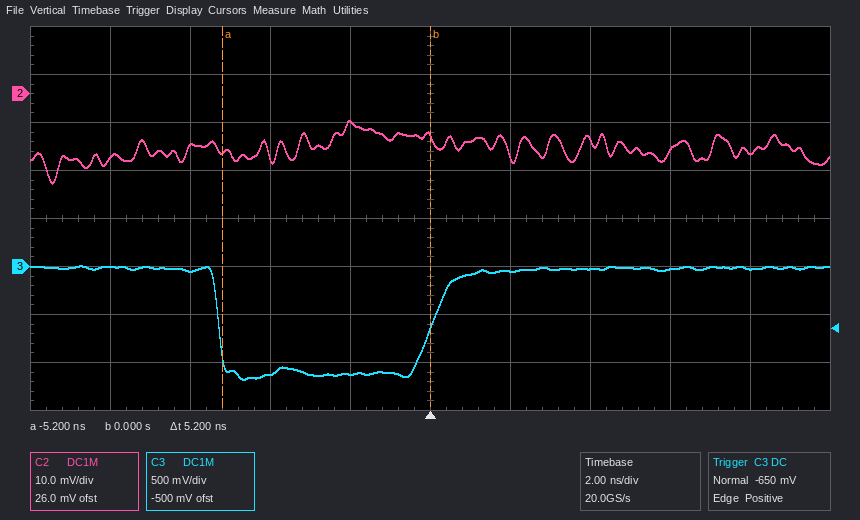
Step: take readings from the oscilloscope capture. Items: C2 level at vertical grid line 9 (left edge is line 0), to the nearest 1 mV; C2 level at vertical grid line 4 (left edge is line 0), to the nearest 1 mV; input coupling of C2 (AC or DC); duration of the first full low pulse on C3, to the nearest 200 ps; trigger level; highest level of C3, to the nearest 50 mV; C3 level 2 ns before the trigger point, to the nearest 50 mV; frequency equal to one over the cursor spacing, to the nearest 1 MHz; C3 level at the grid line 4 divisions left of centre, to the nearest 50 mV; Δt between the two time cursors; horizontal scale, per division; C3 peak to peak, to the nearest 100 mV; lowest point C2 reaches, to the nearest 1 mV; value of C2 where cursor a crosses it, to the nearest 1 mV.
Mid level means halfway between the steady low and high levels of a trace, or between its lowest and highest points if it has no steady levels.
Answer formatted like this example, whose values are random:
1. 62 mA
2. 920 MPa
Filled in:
1. -12 mV
2. -6 mV
3. DC
4. 5.4 ns
5. -650 mV
6. 0 mV
7. -1.10 V
8. 192 MHz
9. 0 mV
10. 5.2 ns
11. 2 ns
12. 1.20 V
13. -19 mV
14. -12 mV
